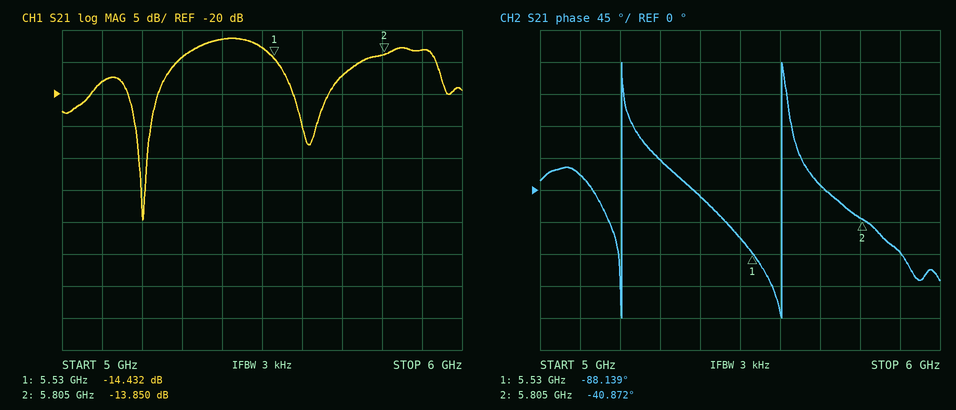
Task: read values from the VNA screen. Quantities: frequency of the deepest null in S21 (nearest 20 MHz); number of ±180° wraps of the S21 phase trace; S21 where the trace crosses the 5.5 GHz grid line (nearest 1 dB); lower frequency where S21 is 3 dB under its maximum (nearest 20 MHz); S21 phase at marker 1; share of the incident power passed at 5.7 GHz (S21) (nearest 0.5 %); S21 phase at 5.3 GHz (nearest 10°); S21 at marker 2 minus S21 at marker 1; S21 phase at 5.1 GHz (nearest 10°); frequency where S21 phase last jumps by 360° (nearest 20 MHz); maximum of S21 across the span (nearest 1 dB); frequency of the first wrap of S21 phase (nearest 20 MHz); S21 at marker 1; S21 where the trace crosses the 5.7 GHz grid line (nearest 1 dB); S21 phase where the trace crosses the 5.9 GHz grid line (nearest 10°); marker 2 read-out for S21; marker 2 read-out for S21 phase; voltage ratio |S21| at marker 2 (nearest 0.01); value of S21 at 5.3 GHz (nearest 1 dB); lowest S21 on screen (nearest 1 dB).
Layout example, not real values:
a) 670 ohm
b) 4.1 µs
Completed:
a) 5.20 GHz
b) 2
c) -13 dB
d) 5.30 GHz
e) -88.139°
f) 2.0 %
g) 40°
h) 0.582 dB
i) 20°
j) 5.60 GHz
k) -11 dB
l) 5.20 GHz
m) -14.432 dB
n) -17 dB
o) -90°
p) -13.850 dB
q) -40.872°
r) 0.20
s) -14 dB
t) -40 dB
